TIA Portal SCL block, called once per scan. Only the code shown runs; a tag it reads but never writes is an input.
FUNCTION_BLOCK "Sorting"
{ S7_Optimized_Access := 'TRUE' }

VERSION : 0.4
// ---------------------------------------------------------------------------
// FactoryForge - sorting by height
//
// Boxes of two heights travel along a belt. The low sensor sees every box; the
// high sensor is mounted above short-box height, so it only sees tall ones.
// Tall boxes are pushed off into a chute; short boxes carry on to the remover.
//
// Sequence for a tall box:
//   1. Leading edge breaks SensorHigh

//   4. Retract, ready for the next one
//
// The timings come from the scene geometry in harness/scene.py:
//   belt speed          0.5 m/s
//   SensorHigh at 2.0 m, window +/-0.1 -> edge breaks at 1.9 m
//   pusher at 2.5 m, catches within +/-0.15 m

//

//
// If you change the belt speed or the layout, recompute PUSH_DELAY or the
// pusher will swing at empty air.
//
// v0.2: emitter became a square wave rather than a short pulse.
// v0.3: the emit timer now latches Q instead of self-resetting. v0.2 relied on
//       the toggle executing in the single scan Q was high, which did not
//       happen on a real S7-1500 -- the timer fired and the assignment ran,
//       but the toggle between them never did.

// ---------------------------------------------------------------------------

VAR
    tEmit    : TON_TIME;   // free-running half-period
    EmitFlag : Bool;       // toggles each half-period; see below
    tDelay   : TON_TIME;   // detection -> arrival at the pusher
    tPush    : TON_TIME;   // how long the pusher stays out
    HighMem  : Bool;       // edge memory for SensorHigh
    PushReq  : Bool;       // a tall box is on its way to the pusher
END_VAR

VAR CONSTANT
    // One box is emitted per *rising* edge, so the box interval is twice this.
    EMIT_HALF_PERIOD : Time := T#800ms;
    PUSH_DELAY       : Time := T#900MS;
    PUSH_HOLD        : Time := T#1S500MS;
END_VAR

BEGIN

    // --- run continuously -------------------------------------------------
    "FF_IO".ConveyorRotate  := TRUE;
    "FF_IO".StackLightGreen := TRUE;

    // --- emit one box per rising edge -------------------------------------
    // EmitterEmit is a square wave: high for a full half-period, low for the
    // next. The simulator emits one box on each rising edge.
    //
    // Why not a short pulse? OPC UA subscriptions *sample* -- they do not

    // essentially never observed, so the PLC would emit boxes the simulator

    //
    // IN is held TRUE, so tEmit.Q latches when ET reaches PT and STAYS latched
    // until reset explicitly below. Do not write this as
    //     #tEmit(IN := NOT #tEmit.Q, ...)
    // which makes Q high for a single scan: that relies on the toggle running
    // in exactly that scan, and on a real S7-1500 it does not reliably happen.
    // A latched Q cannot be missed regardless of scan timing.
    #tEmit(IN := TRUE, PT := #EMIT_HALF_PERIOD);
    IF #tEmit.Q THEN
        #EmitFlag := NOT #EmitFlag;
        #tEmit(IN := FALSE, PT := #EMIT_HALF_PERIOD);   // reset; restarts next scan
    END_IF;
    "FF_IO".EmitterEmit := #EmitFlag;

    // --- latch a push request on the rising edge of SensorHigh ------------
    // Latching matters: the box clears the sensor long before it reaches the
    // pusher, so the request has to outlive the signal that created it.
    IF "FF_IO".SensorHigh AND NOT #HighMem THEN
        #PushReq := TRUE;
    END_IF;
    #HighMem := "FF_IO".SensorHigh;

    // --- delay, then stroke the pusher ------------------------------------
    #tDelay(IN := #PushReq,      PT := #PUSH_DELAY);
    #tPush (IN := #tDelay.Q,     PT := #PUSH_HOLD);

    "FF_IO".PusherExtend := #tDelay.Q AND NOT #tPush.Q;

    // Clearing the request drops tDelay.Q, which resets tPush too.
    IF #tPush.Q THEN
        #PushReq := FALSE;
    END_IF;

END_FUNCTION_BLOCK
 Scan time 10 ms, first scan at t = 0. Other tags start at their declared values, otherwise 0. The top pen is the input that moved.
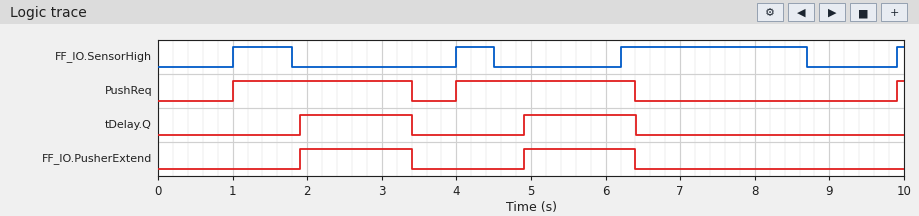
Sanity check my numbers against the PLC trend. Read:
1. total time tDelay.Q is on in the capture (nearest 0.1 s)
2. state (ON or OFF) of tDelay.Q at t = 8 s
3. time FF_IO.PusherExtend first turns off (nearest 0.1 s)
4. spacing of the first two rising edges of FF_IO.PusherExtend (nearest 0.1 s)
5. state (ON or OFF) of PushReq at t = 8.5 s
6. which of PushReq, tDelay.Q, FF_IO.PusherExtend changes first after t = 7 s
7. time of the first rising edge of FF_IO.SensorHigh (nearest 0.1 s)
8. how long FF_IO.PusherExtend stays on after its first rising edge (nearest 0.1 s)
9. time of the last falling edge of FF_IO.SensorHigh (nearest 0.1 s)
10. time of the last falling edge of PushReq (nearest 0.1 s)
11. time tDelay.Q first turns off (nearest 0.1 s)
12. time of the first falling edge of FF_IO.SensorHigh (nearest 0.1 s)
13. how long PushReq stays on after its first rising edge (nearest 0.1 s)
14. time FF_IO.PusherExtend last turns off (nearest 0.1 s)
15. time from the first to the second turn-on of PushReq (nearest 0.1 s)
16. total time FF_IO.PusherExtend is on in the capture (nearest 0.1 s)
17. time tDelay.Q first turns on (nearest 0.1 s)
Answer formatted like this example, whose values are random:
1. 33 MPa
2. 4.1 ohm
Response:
1. 3.0 s
2. OFF
3. 3.4 s
4. 3.0 s
5. OFF
6. PushReq
7. 1.0 s
8. 1.5 s
9. 8.7 s
10. 6.4 s
11. 3.4 s
12. 1.8 s
13. 2.4 s
14. 6.4 s
15. 3.0 s
16. 3.0 s
17. 1.9 s
